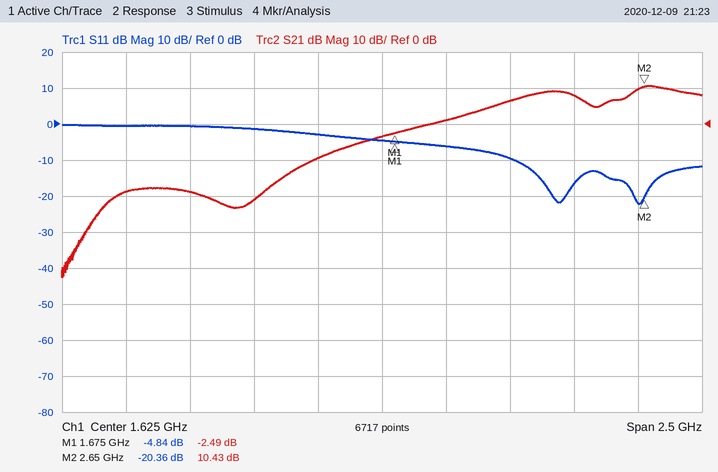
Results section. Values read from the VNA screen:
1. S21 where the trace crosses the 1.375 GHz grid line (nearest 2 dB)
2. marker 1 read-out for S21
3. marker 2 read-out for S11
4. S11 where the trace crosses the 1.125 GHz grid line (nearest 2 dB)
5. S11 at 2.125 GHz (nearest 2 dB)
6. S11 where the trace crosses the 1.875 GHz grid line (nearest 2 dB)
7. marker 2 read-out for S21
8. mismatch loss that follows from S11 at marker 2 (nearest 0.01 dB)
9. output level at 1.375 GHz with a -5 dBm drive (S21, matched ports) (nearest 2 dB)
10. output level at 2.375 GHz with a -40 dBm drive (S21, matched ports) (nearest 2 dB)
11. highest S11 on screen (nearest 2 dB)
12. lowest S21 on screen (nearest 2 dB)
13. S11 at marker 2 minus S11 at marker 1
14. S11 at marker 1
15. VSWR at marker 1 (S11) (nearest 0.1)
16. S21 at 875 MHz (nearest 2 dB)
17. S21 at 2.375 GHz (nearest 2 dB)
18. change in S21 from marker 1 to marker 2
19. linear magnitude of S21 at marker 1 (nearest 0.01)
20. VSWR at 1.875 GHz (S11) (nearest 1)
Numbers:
-10 dB
-2.49 dB
-20.36 dB
-2 dB
-10 dB
-6 dB
10.43 dB
0.04 dB
-14 dBm
-32 dBm
0 dB
-42 dB
-15.52 dB
-4.84 dB
3.7
-18 dB
8 dB
12.92 dB
0.75
3
